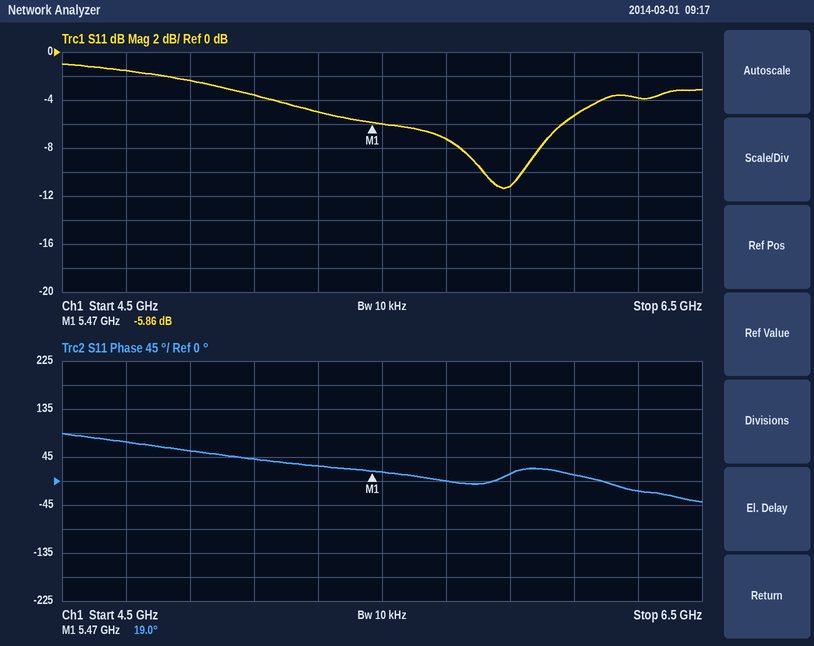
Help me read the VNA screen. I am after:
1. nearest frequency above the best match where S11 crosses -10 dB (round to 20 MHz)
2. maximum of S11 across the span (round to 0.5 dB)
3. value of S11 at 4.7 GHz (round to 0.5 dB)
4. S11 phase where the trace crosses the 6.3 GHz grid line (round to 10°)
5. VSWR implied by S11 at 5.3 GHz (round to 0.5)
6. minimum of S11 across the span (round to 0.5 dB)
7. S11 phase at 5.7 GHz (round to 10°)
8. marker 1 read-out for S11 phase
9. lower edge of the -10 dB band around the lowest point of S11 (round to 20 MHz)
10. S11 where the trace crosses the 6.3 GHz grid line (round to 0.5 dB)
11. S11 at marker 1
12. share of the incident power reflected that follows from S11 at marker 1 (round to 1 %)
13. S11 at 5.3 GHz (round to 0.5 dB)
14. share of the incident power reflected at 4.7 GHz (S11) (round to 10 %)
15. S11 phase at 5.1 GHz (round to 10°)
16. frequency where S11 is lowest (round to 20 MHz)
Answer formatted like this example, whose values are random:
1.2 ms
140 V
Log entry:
5.94 GHz
-1.0 dB
-1.5 dB
-20°
3.5
-11.5 dB
0°
19.0°
5.82 GHz
-4.0 dB
-5.86 dB
26 %
-5.0 dB
70 %
40°
5.88 GHz
